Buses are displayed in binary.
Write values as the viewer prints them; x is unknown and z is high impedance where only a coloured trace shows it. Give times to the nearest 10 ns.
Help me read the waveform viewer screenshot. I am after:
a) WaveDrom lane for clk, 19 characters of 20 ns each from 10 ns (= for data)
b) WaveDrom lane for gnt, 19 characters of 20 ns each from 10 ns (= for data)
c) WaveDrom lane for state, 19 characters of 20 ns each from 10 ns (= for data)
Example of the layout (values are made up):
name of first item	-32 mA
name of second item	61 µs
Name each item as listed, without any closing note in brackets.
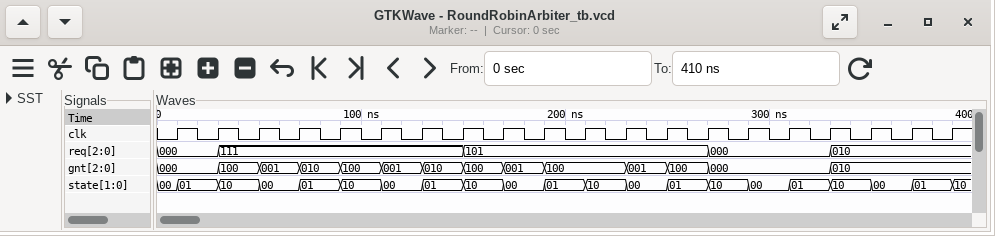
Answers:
WaveDrom lane for clk, 19 characters of 20 ns each from 10 ns	{name: 'clk', wave: 'p..................'}
WaveDrom lane for gnt, 19 characters of 20 ns each from 10 ns	{name: 'gnt', wave: '==========.===..=..', data: '000 100 001 010 100 001 010 100 001 100 001 100 000 010'}
WaveDrom lane for state, 19 characters of 20 ns each from 10 ns	{name: 'state', wave: '===================', data: '01 10 00 01 10 00 01 10 00 01 10 00 01 10 00 01 10 00 01'}
